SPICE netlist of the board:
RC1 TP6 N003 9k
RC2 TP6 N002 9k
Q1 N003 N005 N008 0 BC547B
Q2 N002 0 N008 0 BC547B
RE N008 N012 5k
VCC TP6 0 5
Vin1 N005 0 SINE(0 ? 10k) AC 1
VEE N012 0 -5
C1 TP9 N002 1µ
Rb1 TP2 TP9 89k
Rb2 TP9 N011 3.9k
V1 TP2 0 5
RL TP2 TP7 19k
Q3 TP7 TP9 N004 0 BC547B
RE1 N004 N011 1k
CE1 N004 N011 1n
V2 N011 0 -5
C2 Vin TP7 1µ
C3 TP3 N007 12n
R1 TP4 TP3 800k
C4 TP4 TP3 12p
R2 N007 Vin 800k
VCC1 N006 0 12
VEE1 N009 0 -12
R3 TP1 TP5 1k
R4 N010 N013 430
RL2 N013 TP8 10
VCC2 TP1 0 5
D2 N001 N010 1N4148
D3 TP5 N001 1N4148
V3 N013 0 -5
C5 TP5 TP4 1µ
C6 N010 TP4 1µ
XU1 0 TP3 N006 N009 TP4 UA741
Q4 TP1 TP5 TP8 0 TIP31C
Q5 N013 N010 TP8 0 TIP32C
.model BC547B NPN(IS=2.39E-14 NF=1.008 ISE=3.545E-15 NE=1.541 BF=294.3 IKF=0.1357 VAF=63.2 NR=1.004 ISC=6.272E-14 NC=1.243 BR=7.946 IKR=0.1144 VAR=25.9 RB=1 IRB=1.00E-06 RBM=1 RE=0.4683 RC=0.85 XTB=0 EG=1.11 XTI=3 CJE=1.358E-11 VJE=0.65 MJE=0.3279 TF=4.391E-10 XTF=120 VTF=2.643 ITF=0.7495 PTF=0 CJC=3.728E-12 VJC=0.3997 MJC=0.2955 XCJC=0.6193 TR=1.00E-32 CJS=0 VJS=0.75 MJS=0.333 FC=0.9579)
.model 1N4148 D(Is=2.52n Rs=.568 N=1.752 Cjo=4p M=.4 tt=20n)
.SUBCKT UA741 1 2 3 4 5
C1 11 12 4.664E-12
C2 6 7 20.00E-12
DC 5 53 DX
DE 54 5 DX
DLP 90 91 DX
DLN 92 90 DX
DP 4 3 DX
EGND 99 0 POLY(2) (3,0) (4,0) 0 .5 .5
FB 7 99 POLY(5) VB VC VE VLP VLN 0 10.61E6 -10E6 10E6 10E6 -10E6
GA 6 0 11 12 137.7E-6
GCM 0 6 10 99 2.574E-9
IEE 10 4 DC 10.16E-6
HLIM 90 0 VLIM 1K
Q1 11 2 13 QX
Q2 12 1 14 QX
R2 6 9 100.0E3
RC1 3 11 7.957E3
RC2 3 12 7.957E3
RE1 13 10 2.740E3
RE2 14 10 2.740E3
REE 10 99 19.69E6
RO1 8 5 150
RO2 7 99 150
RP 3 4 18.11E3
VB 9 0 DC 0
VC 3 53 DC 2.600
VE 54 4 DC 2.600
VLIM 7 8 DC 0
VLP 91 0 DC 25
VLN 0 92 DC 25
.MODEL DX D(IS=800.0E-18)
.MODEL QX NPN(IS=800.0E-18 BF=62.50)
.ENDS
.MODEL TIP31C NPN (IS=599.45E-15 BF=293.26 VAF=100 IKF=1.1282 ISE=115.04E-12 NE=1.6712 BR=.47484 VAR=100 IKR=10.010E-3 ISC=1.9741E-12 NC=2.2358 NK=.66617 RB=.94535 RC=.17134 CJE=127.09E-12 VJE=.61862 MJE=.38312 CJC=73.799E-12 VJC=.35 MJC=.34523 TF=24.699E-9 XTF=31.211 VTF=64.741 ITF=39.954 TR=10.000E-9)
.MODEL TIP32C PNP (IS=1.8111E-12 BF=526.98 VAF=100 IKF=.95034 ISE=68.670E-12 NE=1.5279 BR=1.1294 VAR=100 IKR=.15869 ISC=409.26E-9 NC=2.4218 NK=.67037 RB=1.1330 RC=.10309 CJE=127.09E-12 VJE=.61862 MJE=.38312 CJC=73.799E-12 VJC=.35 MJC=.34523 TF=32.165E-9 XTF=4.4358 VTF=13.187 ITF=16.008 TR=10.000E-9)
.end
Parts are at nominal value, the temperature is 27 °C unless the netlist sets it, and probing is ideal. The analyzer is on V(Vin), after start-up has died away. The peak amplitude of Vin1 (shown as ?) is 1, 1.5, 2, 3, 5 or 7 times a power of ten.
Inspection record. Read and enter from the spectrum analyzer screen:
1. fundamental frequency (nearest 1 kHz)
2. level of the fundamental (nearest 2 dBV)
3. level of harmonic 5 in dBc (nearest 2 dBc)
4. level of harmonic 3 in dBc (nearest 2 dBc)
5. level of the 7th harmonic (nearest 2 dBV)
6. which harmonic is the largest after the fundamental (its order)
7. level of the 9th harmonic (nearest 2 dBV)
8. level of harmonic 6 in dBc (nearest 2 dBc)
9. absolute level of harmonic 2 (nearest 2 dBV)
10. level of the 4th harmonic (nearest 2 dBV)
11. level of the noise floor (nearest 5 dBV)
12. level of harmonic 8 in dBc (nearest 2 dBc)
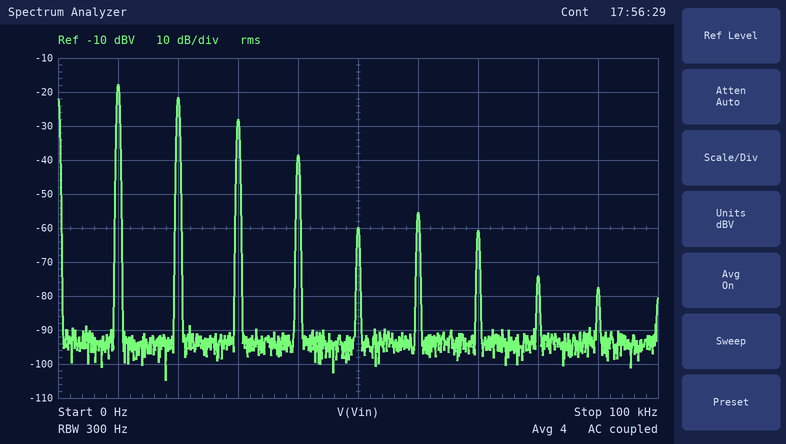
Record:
10 kHz
-18 dBV
-42 dBc
-10 dBc
-60 dBV
2
-78 dBV
-38 dBc
-22 dBV
-38 dBV
-95 dBV
-56 dBc
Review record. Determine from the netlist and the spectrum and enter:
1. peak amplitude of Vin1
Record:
7 mV
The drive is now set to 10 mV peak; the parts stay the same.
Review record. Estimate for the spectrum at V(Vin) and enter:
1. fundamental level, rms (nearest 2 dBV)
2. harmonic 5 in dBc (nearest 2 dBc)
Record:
-10 dBV
-30 dBc
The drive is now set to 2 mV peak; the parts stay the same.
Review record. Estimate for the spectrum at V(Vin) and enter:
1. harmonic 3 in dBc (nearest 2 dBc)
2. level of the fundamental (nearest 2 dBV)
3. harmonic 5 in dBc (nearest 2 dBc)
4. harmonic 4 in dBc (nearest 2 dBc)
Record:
-22 dBc
-42 dBV
-54 dBc
-36 dBc
